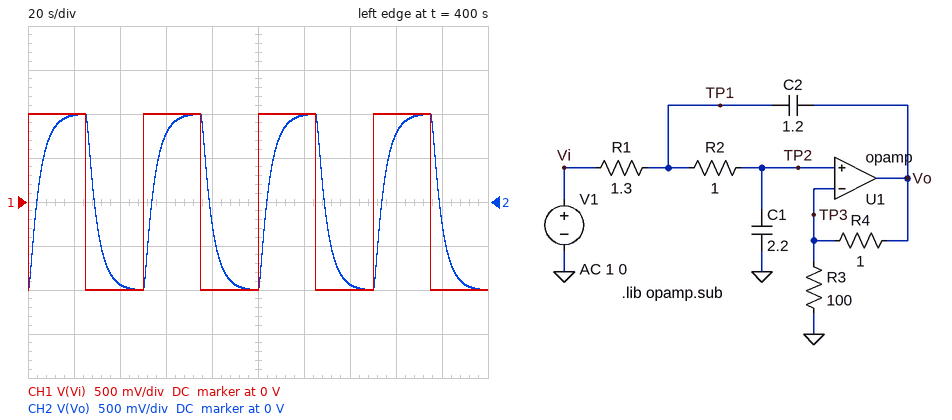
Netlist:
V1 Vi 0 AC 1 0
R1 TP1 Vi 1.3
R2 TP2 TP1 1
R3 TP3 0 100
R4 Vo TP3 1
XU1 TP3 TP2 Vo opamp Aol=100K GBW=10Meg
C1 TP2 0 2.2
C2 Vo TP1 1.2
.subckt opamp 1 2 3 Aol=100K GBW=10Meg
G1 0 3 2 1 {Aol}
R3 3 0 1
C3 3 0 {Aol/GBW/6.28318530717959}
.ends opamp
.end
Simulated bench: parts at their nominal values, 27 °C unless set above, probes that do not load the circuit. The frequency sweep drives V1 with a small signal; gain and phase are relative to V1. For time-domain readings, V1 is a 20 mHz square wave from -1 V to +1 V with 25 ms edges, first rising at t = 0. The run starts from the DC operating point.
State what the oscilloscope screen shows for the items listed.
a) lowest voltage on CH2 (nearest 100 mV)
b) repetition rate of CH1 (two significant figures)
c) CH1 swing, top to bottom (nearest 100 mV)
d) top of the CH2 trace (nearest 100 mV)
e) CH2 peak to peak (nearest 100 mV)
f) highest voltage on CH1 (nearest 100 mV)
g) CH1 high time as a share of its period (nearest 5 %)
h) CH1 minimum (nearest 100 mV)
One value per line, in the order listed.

-1.0 V
20 mHz
2.0 V
1.0 V
2.0 V
1.0 V
50 %
-1.0 V
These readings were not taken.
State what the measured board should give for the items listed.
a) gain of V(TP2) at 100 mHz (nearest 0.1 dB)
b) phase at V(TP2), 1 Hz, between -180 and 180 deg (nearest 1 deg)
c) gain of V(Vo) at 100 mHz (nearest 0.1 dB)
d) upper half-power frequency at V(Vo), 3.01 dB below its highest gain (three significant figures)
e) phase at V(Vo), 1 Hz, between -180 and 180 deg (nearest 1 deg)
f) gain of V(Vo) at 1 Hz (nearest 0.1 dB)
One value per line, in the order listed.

-10.1 dB
-167 deg
-10.0 dB
36.3 mHz
-167 deg
-42.7 dB
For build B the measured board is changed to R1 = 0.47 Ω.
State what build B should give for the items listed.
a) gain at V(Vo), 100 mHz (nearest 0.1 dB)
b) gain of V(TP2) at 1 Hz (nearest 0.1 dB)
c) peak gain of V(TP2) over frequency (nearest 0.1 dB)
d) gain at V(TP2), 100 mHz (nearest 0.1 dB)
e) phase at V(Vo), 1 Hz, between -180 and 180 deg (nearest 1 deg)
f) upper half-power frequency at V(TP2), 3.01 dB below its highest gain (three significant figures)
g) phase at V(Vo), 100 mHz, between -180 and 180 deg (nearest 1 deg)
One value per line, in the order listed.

-6.3 dB
-34.3 dB
0 dB
-6.4 dB
-157 deg
55.8 mHz
-76 deg
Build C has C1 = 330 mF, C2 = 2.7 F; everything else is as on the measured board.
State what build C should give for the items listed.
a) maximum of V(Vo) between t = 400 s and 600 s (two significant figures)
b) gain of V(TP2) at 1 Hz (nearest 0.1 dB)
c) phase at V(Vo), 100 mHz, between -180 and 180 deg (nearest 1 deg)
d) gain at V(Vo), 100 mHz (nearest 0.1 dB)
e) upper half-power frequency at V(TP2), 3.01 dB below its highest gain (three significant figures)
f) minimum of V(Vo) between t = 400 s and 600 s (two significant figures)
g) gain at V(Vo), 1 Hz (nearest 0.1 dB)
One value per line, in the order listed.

1.7 V
-33.1 dB
-40 deg
3.1 dB
175 mHz
-1.7 V
-33.0 dB
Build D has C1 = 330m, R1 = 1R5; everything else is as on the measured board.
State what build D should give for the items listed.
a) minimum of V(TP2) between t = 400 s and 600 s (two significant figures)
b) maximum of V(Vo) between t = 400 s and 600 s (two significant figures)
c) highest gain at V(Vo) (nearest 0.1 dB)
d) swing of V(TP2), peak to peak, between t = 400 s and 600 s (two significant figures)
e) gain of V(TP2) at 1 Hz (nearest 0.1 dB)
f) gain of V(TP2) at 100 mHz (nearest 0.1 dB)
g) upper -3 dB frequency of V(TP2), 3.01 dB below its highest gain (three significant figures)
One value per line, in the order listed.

-1.3 V
1.3 V
1.1 dB
2.6 V
-27.2 dB
0.7 dB
239 mHz
